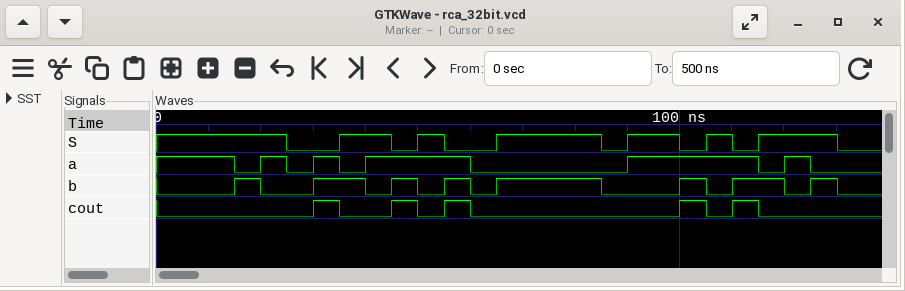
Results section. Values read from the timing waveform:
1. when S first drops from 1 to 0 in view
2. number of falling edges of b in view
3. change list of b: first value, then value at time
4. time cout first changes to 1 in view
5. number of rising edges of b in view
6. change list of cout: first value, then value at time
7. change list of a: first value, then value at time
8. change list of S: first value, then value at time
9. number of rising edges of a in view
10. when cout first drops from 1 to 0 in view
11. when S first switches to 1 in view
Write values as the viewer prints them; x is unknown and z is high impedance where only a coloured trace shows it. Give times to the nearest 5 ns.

25 ns
8
0, 1 at 15 ns, 0 at 20 ns, 1 at 30 ns, 0 at 40 ns, 1 at 45 ns, 0 at 50 ns, 1 at 55 ns, 0 at 60 ns, 1 at 65 ns, 0 at 85 ns, 1 at 100 ns, 0 at 105 ns, 1 at 110 ns, 0 at 120 ns, 1 at 125 ns, 0 at 130 ns
30 ns
8
0, 1 at 30 ns, 0 at 35 ns, 1 at 45 ns, 0 at 50 ns, 1 at 55 ns, 0 at 60 ns, 1 at 100 ns, 0 at 105 ns, 1 at 110 ns, 0 at 115 ns
1, 0 at 15 ns, 1 at 20 ns, 0 at 25 ns, 1 at 30 ns, 0 at 35 ns, 1 at 40 ns, 0 at 60 ns, 1 at 90 ns, 0 at 115 ns, 1 at 120 ns, 0 at 125 ns
1, 0 at 25 ns, 1 at 35 ns, 0 at 45 ns, 1 at 50 ns, 0 at 55 ns, 1 at 65 ns, 0 at 85 ns, 1 at 90 ns, 0 at 100 ns, 1 at 105 ns, 0 at 110 ns, 1 at 115 ns, 0 at 130 ns
5
35 ns
35 ns
